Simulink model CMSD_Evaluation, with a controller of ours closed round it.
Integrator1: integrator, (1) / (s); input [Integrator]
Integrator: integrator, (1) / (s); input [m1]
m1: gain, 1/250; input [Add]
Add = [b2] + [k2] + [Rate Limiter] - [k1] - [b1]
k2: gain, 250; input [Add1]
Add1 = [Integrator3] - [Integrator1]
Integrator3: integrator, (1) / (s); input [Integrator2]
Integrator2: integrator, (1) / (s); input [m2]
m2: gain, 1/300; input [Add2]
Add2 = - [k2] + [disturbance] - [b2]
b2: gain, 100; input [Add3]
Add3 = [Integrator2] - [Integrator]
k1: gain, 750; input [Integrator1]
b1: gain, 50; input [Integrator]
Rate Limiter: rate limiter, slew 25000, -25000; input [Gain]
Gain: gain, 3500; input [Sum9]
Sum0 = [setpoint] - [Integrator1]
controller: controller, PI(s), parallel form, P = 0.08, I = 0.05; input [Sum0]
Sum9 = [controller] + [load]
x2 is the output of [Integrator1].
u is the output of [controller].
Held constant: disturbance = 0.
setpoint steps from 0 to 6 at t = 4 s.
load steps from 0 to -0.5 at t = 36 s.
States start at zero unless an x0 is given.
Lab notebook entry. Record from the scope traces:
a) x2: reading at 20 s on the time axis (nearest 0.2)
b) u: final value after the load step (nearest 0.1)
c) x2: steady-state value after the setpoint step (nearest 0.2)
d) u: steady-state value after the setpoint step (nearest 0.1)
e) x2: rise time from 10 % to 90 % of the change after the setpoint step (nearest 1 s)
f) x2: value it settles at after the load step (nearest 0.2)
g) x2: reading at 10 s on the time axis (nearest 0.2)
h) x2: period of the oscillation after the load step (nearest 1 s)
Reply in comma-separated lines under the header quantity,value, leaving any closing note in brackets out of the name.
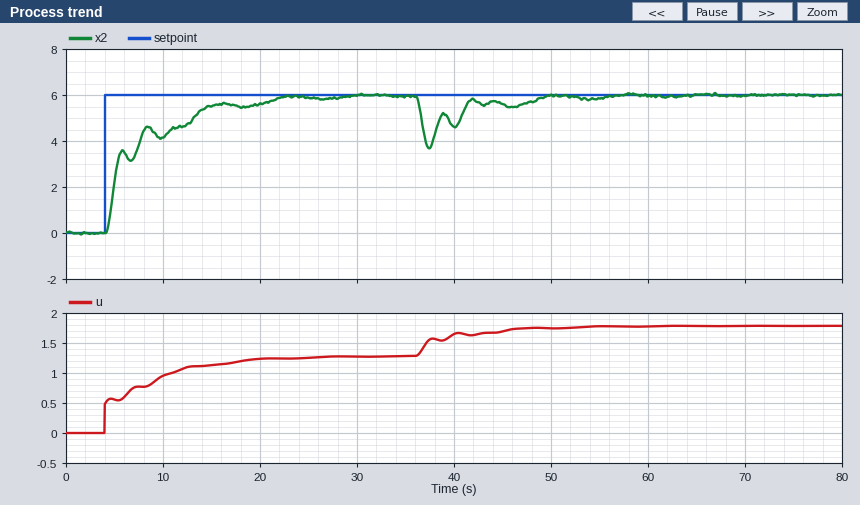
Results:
quantity,value
x2: reading at 20 s on the time axis,5.6
u: final value after the load step,1.8
x2: steady-state value after the setpoint step,6.0
u: steady-state value after the setpoint step,1.3
x2: rise time from 10 % to 90 % of the change after the setpoint step,10 s
x2: value it settles at after the load step,6.0
x2: reading at 10 s on the time axis,4.2
x2: period of the oscillation after the load step,3 s
